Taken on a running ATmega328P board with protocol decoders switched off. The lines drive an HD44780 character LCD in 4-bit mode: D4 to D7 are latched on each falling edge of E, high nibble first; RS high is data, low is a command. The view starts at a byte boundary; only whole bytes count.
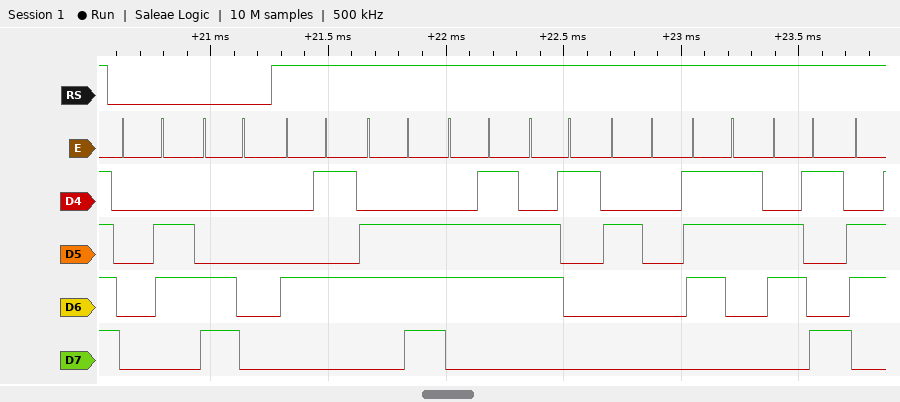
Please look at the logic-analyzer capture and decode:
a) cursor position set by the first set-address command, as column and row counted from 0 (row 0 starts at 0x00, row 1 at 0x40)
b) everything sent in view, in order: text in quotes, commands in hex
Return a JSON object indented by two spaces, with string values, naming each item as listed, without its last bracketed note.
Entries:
{
  "cursor position set by the first set-address command, as column and row counted from 0": "column 0, row 1",
  "everything sent in view, in order: text in quotes, commands in hex": "0x06 0xC0 \"Enga si\""
}
